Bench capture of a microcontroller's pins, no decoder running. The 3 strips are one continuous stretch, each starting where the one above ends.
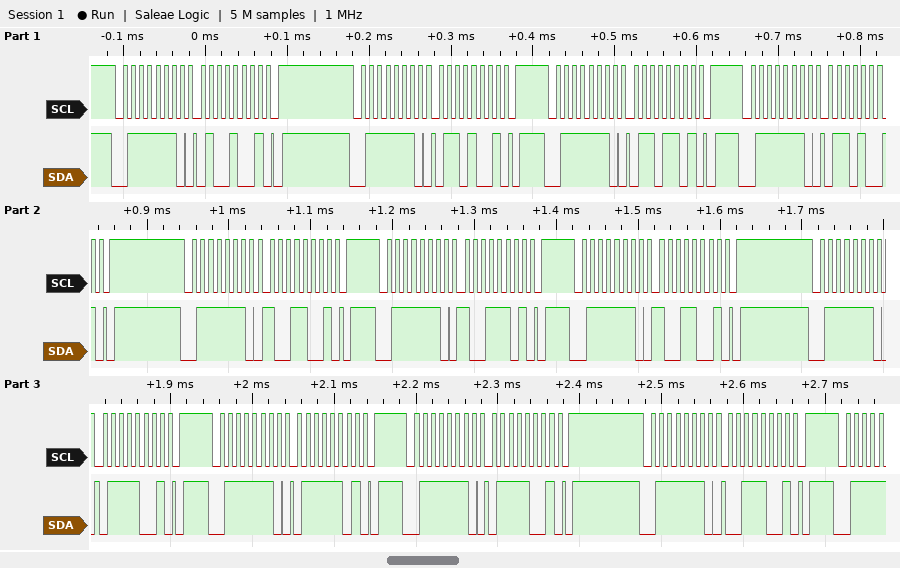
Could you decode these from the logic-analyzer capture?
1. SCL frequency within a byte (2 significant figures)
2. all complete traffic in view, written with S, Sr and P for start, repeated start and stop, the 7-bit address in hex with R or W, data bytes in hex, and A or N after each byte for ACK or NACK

100 kHz
S 3FW A 49 A P S 3FW A 69 A P S 3FW A 6D A P S 3FW A 69 A P S 3FW A 99 A P S 3FW A 9D A P S 3FW A 99 A P S 3FW A 79 A P S 3FW A 7D A P S 3FW A 79 A P S 3FW A 39 A P
